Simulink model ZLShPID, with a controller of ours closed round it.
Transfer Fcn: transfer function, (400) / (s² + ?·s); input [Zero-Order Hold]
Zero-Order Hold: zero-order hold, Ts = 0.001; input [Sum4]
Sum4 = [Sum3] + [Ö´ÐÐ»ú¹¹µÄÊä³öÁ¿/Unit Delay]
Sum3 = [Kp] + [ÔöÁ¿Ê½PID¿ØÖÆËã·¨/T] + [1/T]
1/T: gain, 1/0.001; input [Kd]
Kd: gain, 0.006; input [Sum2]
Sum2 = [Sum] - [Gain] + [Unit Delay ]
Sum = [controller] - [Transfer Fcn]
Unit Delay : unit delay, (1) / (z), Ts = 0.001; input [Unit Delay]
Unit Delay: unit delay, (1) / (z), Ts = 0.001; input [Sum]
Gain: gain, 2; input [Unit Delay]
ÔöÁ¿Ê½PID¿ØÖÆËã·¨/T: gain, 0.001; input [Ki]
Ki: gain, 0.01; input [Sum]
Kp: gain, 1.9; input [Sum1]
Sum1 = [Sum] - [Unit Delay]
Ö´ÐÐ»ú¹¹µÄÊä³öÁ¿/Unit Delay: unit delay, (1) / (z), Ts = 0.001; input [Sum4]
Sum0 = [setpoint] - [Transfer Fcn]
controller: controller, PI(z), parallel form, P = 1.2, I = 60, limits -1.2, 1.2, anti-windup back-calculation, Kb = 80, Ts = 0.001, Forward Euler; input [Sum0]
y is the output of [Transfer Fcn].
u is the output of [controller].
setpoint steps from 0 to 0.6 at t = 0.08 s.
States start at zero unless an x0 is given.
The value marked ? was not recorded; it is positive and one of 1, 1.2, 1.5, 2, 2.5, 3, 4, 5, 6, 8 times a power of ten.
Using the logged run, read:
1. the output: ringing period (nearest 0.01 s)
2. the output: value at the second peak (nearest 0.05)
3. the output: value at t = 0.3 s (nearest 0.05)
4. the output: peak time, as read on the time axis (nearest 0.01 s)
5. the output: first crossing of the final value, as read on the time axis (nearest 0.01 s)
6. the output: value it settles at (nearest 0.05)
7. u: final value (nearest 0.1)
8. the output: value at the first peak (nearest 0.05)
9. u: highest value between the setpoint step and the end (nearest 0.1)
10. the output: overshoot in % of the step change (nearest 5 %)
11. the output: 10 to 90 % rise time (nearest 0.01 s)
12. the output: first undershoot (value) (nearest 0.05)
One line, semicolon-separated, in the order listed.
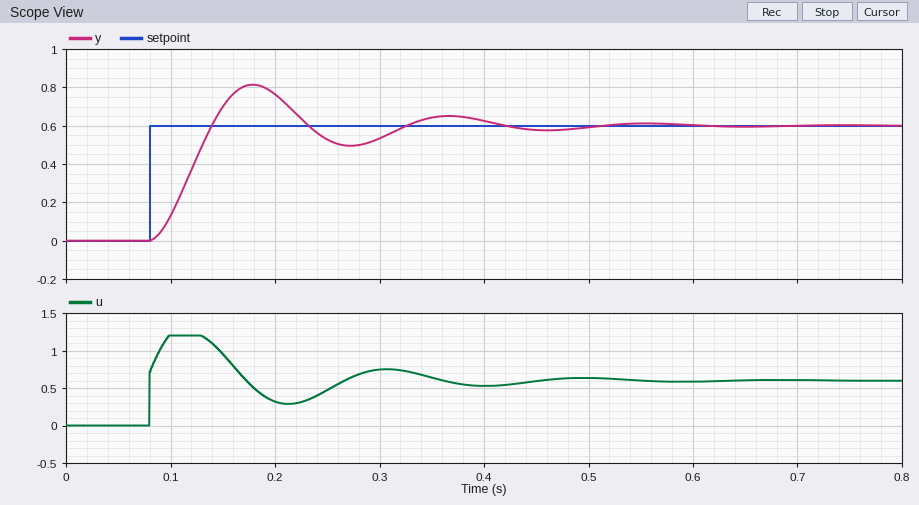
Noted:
0.19 s; 0.65; 0.55; 0.18 s; 0.14 s; 0.60; 0.6; 0.80; 1.2; 35 %; 0.04 s; 0.50
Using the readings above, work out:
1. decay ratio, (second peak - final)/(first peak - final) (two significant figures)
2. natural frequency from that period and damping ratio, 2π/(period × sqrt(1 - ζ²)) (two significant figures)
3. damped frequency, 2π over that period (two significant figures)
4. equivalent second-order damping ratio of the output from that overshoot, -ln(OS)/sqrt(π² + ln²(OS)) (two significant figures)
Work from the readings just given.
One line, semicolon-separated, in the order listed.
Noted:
0.25; 35 rad/s; 33 rad/s; 0.32
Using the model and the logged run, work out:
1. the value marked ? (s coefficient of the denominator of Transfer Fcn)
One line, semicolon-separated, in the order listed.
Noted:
50
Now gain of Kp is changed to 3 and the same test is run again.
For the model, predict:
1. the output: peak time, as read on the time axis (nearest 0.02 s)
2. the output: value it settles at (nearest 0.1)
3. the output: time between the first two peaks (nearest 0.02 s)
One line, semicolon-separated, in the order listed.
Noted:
0.16 s; 0.6; 0.14 s
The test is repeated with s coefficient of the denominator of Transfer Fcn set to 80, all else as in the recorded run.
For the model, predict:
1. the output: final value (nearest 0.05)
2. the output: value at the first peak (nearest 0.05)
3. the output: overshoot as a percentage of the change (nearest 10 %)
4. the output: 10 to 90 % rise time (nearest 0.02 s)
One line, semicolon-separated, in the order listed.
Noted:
0.60; 0.75; 30 %; 0.06 s
